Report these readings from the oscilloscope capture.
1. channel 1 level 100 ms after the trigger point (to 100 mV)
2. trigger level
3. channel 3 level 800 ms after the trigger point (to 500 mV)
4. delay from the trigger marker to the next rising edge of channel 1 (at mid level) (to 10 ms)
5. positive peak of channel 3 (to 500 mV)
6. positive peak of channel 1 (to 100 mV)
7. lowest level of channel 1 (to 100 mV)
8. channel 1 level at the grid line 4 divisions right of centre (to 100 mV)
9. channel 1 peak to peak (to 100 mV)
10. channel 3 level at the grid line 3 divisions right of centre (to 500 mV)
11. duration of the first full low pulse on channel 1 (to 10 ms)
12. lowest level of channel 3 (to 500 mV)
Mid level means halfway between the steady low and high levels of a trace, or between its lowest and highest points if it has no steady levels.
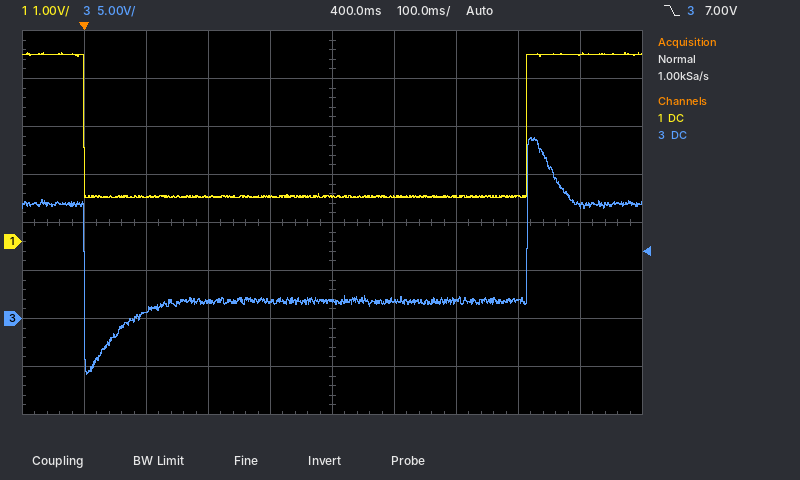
900 mV
7.00 V
12.0 V
710 ms
19.0 V
3.9 V
900 mV
3.9 V
3.0 V
2.0 V
710 ms
-6.0 V
